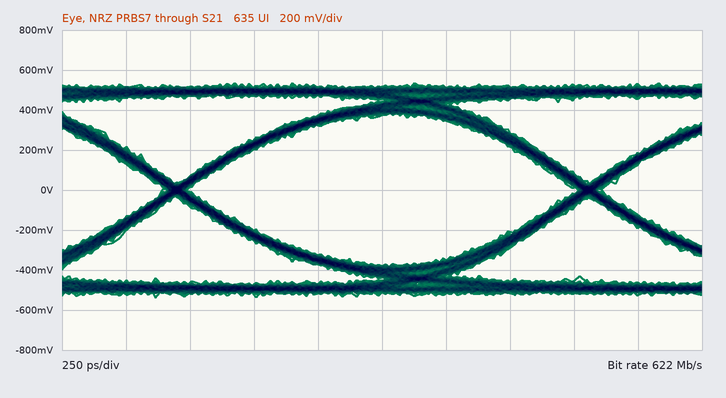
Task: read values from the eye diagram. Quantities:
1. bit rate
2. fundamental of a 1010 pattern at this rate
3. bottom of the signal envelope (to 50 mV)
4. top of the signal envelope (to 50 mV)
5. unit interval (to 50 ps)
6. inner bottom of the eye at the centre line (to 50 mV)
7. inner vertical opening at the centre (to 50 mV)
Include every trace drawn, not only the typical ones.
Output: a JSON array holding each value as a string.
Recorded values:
["622 Mb/s", "311 MHz", "-550 mV", "550 mV", "1.60 ns", "-400 mV", "750 mV"]
